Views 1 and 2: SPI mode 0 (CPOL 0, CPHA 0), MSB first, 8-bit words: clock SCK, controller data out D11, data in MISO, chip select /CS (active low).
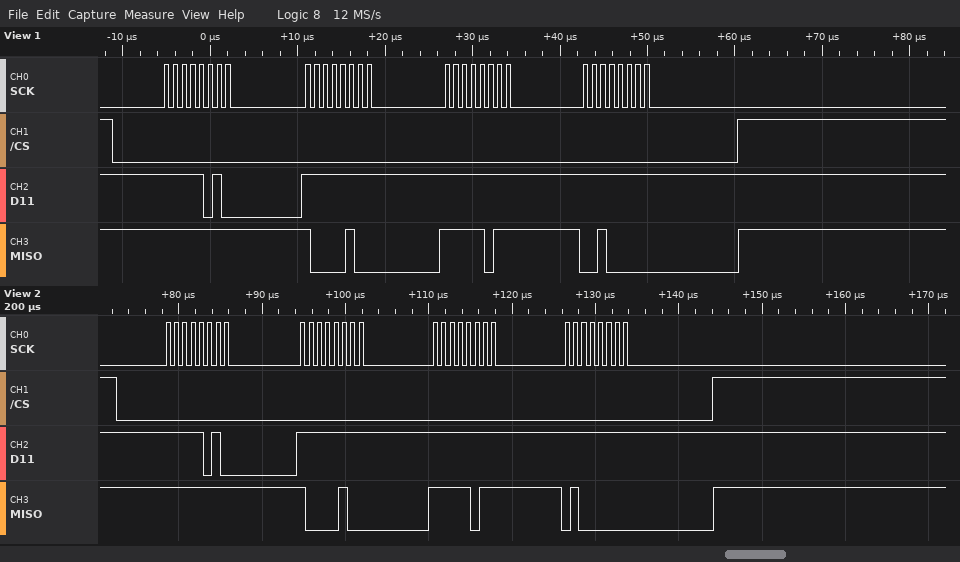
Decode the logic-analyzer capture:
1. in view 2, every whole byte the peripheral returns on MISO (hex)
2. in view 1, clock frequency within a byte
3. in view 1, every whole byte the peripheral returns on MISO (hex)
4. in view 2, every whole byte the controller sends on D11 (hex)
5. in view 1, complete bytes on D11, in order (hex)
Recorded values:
0xFF 0x84 0xFB 0x40
1 MHz
FF 84 FB 20
0xFA 0xFF 0xFF 0xFF
FA FF FF FF
